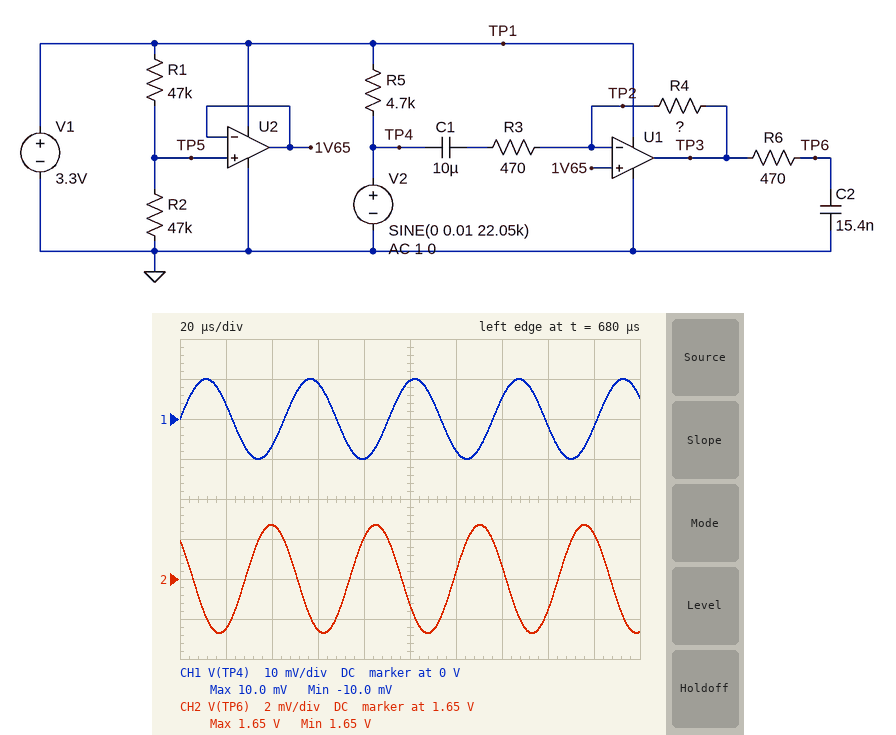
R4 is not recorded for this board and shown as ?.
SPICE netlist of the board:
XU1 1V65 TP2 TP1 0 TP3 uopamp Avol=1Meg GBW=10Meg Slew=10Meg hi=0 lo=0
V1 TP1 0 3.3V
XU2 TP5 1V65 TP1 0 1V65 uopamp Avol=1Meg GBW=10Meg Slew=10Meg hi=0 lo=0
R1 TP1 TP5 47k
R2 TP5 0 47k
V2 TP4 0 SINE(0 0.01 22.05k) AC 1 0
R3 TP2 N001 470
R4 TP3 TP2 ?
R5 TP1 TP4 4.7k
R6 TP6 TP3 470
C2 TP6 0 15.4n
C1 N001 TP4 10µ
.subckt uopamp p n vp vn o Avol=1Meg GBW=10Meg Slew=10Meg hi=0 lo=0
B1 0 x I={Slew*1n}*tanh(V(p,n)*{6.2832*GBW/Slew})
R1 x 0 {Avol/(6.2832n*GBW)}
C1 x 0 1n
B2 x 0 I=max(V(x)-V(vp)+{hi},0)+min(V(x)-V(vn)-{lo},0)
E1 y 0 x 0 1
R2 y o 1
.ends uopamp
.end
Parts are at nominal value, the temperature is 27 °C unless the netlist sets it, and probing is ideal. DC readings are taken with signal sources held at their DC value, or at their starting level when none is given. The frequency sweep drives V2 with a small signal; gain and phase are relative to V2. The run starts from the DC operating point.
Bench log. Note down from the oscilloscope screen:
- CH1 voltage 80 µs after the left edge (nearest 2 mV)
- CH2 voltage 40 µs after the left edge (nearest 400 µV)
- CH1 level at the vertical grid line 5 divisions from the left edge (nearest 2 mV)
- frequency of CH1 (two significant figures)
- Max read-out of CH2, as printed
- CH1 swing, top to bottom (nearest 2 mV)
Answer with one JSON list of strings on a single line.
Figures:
["-10 mV", "1.6528 V", "10 mV", "22 kHz", "1.65 V", "20 mV"]
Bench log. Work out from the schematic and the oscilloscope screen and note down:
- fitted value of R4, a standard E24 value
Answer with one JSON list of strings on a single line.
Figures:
["180 Ω"]
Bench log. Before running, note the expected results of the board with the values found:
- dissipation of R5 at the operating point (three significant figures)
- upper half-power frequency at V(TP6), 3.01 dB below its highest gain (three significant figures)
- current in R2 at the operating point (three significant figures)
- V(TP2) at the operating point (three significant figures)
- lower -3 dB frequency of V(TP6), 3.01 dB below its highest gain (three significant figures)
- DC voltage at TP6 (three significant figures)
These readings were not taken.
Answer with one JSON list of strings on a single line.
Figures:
["2.32 mW", "22.1 kHz", "35.1 µA", "1.65 V", "33.8 Hz", "1.65 V"]
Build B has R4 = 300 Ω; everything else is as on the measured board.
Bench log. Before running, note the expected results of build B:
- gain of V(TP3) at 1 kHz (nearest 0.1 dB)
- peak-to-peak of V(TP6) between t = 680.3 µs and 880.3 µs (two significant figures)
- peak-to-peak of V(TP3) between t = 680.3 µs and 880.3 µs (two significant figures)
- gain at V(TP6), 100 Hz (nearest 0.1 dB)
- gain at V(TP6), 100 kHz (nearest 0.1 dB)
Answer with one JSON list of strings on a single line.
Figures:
["-3.9 dB", "9.0 mV", "13 mV", "-4.4 dB", "-17.3 dB"]
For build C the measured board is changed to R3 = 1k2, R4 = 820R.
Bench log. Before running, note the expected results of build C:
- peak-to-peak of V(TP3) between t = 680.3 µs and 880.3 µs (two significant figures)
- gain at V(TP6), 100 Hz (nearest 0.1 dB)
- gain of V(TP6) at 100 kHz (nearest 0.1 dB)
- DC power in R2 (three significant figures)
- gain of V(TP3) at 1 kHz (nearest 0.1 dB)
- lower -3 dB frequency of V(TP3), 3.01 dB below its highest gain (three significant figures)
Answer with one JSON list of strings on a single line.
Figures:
["14 mV", "-3.4 dB", "-16.7 dB", "57.9 µW", "-3.3 dB", "13.3 Hz"]
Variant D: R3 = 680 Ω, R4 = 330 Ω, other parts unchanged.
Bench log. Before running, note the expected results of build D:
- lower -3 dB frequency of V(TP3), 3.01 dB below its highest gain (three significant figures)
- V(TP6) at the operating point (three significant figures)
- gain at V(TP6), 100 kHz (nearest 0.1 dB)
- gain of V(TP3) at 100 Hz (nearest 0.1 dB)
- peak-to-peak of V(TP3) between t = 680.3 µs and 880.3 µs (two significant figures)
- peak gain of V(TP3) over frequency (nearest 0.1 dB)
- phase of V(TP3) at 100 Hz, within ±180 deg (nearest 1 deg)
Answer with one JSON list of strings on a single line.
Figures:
["23.4 Hz", "1.65 V", "-19.6 dB", "-6.5 dB", "9.7 mV", "-6.3 dB", "-167 deg"]
